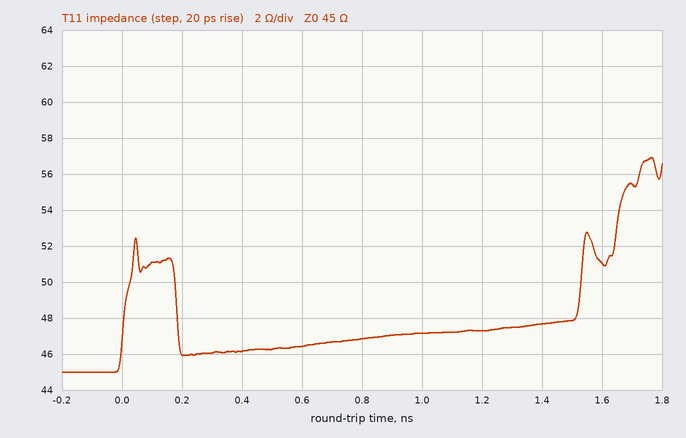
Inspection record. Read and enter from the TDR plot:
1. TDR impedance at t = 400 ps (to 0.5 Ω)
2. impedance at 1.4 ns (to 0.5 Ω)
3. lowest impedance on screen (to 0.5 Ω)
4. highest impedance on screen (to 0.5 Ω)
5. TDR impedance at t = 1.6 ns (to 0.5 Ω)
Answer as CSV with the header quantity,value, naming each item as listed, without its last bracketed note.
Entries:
quantity,value
TDR impedance at t = 400 ps,46.0 Ω
impedance at 1.4 ns,47.5 Ω
lowest impedance on screen,45.0 Ω
highest impedance on screen,57.0 Ω
TDR impedance at t = 1.6 ns,51.0 Ω
